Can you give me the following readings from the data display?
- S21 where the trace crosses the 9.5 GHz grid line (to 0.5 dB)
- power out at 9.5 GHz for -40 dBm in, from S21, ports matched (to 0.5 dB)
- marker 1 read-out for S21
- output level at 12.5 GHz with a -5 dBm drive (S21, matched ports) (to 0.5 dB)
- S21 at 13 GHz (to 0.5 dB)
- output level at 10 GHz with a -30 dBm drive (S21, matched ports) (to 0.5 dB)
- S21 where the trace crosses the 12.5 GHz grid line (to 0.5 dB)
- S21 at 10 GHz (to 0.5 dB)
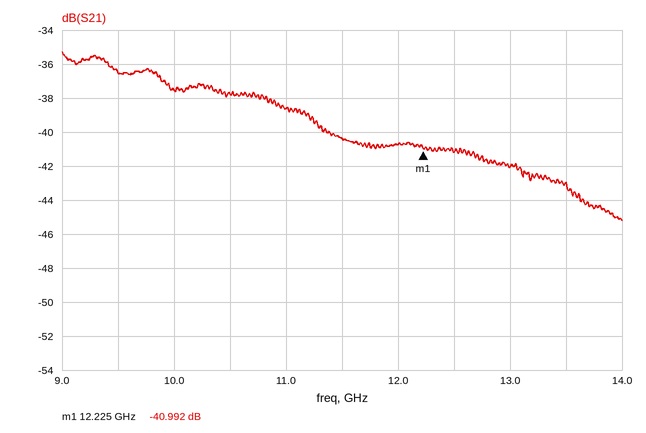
-36.5 dB
-76.5 dBm
-40.992 dB
-46.0 dBm
-42.0 dB
-67.5 dBm
-41.0 dB
-37.5 dB
